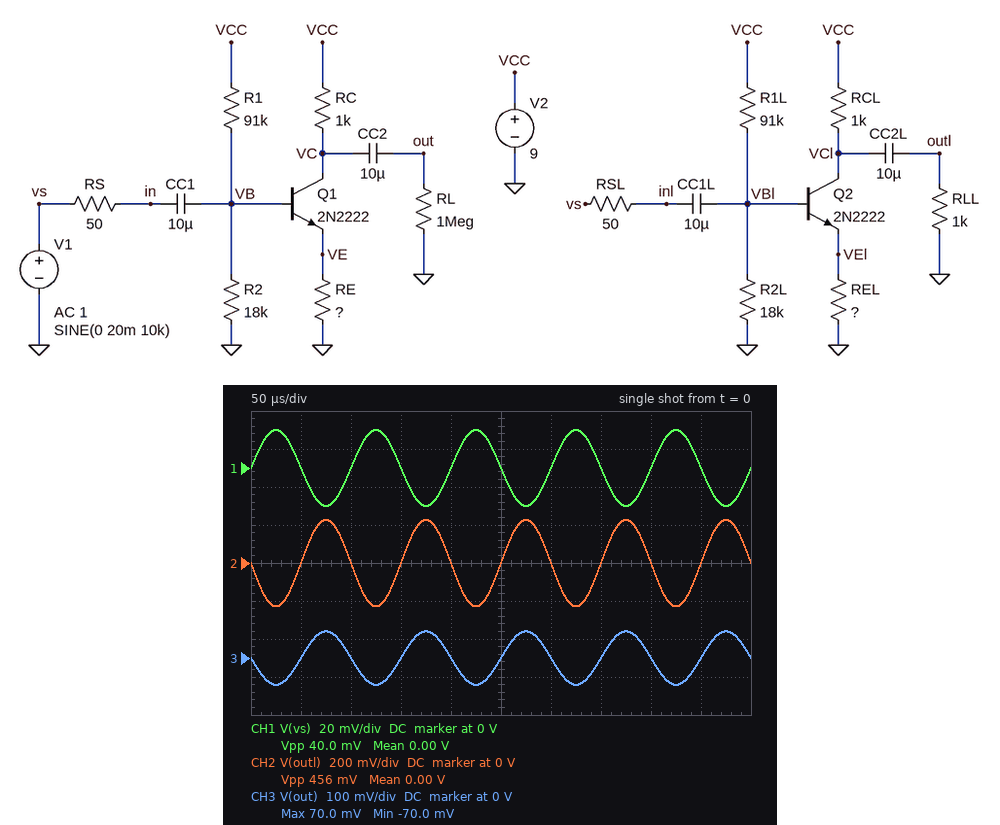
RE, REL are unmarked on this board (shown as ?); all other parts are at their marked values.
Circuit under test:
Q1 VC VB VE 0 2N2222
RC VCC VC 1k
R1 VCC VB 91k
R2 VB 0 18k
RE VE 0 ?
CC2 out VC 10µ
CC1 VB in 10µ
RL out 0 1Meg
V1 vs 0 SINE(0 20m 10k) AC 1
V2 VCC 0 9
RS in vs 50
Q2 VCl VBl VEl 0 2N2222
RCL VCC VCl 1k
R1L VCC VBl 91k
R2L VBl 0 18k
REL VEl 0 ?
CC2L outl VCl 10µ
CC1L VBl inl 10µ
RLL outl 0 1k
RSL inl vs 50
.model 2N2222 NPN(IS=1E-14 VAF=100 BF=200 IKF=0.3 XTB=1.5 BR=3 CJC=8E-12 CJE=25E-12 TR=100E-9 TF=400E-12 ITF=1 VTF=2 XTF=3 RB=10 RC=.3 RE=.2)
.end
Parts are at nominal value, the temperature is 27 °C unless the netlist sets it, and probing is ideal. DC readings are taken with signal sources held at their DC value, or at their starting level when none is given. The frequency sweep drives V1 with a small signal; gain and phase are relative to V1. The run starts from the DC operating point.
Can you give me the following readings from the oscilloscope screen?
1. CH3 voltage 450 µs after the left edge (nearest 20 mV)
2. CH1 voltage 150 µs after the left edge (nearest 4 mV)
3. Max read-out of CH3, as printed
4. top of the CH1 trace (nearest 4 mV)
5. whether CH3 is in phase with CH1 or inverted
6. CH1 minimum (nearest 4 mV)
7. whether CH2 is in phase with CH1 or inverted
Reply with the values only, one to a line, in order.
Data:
0 V
0 V
70.0 mV
20 mV
inverted
-20 mV
inverted
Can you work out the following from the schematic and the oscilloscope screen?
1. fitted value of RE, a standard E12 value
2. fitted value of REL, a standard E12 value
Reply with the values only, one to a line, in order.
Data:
270 Ω
39 Ω
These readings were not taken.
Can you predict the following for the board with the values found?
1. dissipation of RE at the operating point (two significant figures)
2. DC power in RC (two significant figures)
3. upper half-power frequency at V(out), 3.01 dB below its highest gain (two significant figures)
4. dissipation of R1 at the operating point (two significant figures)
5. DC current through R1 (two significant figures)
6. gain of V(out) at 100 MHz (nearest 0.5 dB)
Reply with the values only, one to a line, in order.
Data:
1.5 mW
5.6 mW
33 MHz
650 µW
84 µA
3.0 dB
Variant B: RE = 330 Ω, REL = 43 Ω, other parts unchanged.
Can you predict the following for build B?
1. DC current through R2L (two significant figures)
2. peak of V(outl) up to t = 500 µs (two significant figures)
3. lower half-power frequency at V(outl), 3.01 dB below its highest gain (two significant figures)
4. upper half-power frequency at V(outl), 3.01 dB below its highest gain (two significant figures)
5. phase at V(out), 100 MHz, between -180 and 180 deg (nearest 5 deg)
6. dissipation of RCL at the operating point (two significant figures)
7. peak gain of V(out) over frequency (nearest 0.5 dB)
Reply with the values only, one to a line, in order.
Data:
55 µA
210 mV
8.8 Hz
22 MHz
50 deg
43 mW
9.0 dB
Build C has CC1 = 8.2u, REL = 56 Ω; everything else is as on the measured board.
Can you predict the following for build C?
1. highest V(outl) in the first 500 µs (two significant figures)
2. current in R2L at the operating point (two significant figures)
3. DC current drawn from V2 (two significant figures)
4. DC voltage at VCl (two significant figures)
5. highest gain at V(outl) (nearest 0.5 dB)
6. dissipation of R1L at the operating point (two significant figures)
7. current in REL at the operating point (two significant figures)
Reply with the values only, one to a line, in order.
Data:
160 mV
58 µA
8.5 mA
3.0 V
18.0 dB
700 µW
6.0 mA
